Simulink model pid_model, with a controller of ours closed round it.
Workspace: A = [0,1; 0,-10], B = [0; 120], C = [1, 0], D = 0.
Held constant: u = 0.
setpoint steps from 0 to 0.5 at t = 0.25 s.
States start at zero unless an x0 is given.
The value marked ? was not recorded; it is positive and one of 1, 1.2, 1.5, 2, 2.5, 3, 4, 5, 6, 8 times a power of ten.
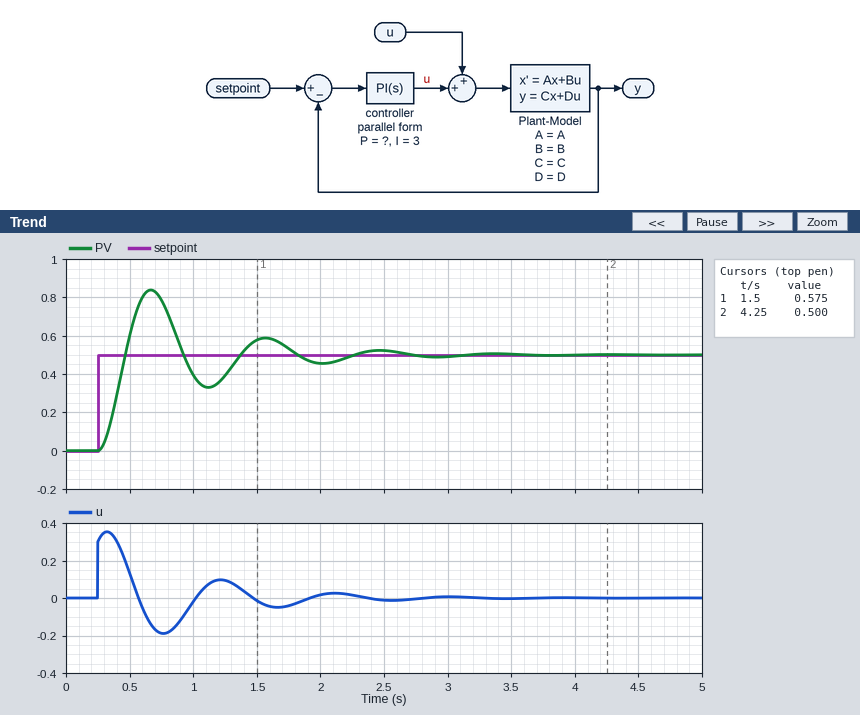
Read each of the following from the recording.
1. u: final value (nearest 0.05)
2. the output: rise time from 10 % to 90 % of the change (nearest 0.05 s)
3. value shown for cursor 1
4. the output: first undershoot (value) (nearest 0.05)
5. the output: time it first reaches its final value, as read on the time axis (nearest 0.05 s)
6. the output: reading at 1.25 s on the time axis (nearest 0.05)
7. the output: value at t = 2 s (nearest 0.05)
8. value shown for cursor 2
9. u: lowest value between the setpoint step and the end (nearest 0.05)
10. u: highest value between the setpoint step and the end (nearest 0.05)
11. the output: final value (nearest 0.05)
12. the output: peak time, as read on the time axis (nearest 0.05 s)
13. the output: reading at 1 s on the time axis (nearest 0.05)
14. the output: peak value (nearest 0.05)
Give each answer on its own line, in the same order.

0.00
0.15 s
0.575
0.35
0.45 s
0.40
0.45
0.500
-0.20
0.35
0.50
0.65 s
0.40
0.85
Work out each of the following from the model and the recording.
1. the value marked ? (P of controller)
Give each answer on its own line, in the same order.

0.6
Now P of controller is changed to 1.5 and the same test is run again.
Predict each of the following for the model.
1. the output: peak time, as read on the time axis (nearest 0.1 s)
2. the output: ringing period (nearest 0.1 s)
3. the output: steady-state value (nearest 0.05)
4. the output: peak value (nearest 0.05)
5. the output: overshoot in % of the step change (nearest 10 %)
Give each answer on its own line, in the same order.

0.5 s
0.5 s
0.50
0.75
50 %
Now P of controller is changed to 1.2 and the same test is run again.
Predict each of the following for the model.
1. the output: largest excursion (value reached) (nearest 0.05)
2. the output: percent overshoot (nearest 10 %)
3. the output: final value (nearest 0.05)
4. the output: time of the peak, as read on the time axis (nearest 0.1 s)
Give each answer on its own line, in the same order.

0.75
50 %
0.50
0.5 s
